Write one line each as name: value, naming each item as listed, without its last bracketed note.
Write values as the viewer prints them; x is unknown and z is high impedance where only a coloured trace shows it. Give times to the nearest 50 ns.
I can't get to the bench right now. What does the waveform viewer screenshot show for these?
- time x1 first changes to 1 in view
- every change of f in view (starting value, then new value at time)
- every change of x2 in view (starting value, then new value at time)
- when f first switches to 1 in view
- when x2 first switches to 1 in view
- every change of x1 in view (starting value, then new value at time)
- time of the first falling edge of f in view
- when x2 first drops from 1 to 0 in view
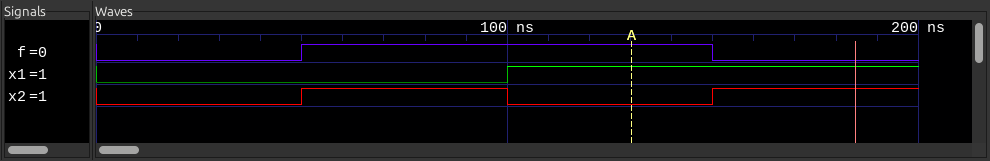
time x1 first changes to 1 in view: 100 ns
every change of f in view: 0, 1 at 50 ns, 0 at 150 ns
every change of x2 in view: 0, 1 at 50 ns, 0 at 100 ns, 1 at 150 ns
when f first switches to 1 in view: 50 ns
when x2 first switches to 1 in view: 50 ns
every change of x1 in view: 0, 1 at 100 ns
time of the first falling edge of f in view: 150 ns
when x2 first drops from 1 to 0 in view: 100 ns
